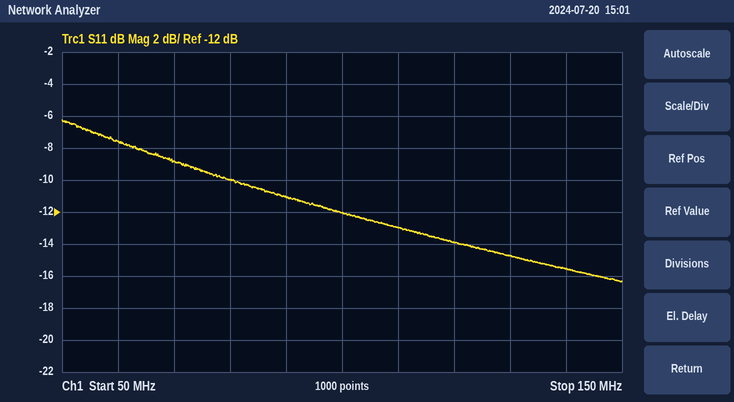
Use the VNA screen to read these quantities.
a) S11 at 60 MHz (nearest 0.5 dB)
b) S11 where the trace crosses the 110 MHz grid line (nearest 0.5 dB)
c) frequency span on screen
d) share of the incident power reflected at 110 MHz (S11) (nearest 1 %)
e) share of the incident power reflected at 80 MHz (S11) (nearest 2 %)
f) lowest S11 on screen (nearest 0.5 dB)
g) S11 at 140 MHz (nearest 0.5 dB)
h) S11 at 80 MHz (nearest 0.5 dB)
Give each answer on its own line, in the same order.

-7.5 dB
-13.0 dB
100 MHz
5 %
10 %
-16.5 dB
-15.5 dB
-10.0 dB
